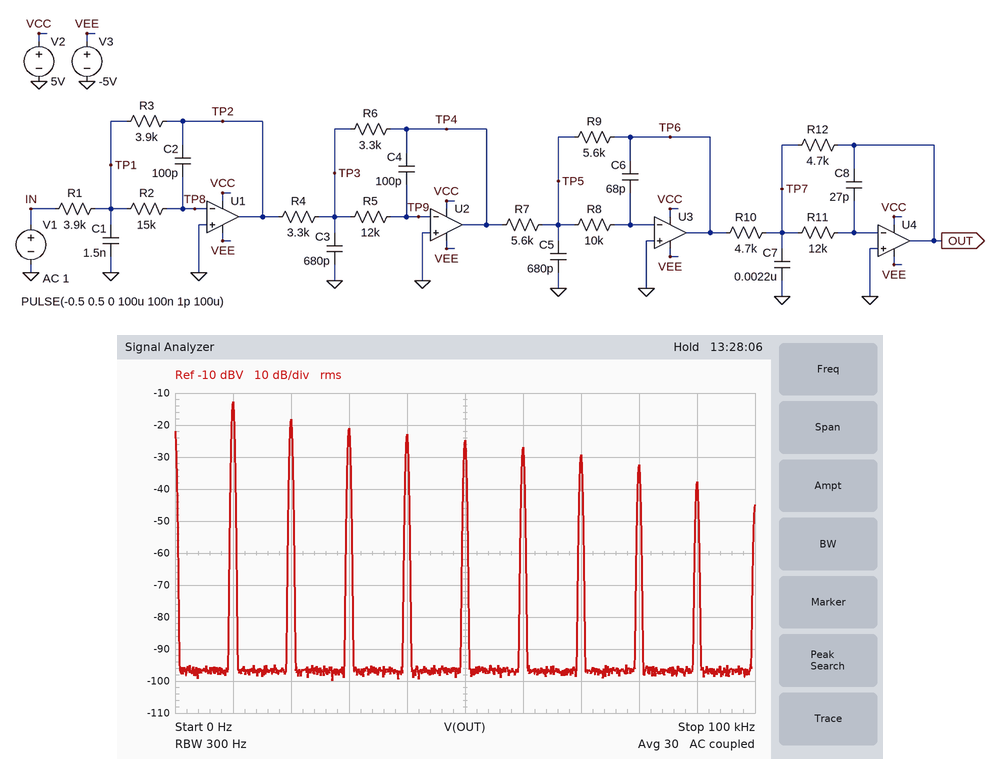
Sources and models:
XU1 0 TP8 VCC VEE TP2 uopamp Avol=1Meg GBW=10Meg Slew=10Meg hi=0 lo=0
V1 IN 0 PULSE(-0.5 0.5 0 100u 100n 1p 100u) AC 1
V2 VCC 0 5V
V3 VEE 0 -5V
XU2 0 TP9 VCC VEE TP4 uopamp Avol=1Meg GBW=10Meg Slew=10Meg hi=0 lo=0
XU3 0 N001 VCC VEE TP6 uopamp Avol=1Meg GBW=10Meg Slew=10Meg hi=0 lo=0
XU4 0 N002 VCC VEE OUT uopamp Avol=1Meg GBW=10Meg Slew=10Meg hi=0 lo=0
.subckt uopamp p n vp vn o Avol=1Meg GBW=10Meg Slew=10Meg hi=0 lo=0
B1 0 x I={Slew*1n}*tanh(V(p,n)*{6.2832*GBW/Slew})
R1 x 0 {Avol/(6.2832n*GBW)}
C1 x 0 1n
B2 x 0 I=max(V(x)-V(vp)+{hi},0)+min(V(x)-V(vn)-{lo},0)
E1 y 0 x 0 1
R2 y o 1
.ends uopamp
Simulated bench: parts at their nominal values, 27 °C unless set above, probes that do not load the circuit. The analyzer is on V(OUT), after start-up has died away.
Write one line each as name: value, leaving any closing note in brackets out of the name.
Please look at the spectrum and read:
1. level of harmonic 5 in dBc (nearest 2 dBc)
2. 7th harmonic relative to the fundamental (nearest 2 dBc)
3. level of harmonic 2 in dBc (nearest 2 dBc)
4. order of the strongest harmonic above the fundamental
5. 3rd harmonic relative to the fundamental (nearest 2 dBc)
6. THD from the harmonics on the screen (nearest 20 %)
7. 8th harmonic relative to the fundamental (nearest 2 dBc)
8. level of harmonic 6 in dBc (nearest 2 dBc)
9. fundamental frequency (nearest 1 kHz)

level of harmonic 5 in dBc: -12 dBc
7th harmonic relative to the fundamental: -16 dBc
level of harmonic 2 in dBc: -6 dBc
order of the strongest harmonic above the fundamental: 2
3rd harmonic relative to the fundamental: -8 dBc
THD from the harmonics on the screen: 80 %
8th harmonic relative to the fundamental: -20 dBc
level of harmonic 6 in dBc: -14 dBc
fundamental frequency: 10 kHz
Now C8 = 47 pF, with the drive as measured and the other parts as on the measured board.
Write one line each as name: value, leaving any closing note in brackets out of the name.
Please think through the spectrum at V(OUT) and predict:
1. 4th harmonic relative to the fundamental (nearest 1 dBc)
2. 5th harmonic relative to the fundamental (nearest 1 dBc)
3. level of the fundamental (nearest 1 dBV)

4th harmonic relative to the fundamental: -9 dBc
5th harmonic relative to the fundamental: -11 dBc
level of the fundamental: -13 dBV
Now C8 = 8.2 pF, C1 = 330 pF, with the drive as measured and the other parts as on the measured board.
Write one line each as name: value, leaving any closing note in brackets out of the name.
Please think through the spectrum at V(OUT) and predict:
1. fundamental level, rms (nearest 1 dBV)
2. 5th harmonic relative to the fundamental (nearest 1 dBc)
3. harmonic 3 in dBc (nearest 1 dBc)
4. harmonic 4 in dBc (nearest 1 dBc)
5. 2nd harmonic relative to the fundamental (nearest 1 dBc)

fundamental level, rms: -13 dBV
5th harmonic relative to the fundamental: -16 dBc
harmonic 3 in dBc: -10 dBc
harmonic 4 in dBc: -13 dBc
2nd harmonic relative to the fundamental: -6 dBc
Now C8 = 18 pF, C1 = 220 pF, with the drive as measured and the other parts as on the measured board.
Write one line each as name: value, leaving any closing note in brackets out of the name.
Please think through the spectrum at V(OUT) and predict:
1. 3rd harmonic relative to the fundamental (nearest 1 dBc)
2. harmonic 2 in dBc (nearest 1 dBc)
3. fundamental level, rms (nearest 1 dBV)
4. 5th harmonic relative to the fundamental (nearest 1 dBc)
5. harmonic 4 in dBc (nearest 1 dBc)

3rd harmonic relative to the fundamental: -10 dBc
harmonic 2 in dBc: -6 dBc
fundamental level, rms: -13 dBV
5th harmonic relative to the fundamental: -15 dBc
harmonic 4 in dBc: -13 dBc
